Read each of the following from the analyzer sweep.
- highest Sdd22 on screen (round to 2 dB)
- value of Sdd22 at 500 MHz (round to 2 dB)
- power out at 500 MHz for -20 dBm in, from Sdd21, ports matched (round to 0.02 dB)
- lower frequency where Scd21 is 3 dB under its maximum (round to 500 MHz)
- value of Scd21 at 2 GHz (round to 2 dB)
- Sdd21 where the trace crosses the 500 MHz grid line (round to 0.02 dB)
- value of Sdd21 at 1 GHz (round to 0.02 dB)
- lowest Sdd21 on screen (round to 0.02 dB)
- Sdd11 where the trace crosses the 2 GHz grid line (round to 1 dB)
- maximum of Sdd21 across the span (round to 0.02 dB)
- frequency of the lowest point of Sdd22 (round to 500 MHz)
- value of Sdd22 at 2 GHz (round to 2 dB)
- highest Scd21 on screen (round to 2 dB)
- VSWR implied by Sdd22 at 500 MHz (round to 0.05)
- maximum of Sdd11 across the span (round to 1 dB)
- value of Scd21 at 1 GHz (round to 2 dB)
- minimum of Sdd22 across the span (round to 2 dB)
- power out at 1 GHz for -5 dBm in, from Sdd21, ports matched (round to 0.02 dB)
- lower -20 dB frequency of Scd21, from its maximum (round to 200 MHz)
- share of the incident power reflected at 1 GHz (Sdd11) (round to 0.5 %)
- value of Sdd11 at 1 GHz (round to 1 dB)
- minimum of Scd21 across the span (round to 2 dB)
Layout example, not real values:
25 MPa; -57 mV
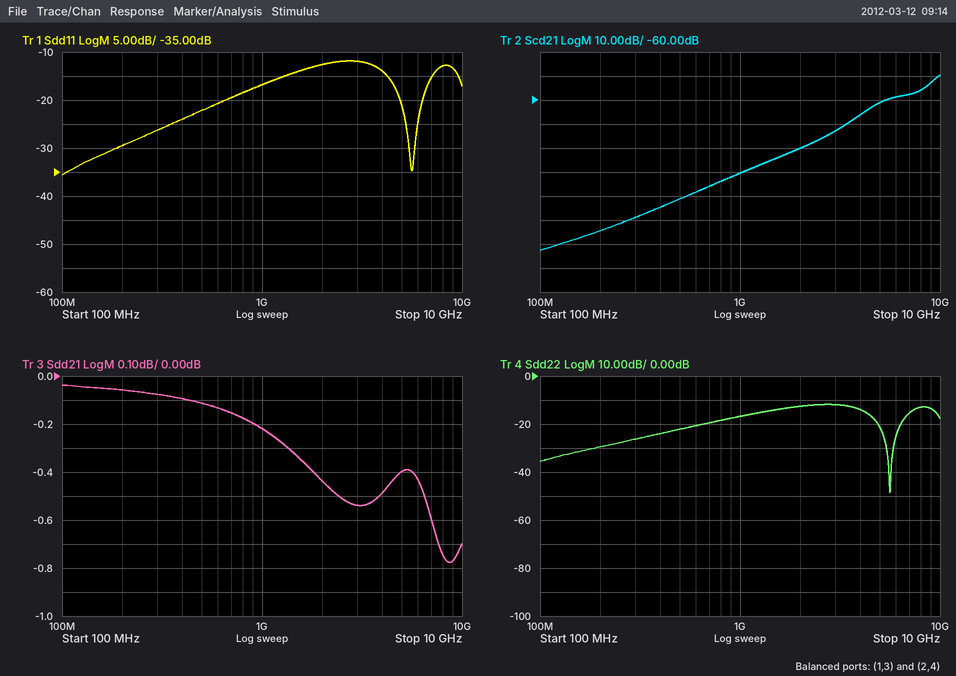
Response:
-12 dB; -22 dB; -20.12 dBm; 9.0 GHz; -80 dB; -0.12 dB; -0.22 dB; -0.78 dB; -13 dB; -0.04 dB; 5.5 GHz; -12 dB; -50 dB; 1.15; -12 dB; -90 dB; -48 dB; -5.22 dBm; 3.4 GHz; 2.0 %; -17 dB; -122 dB
